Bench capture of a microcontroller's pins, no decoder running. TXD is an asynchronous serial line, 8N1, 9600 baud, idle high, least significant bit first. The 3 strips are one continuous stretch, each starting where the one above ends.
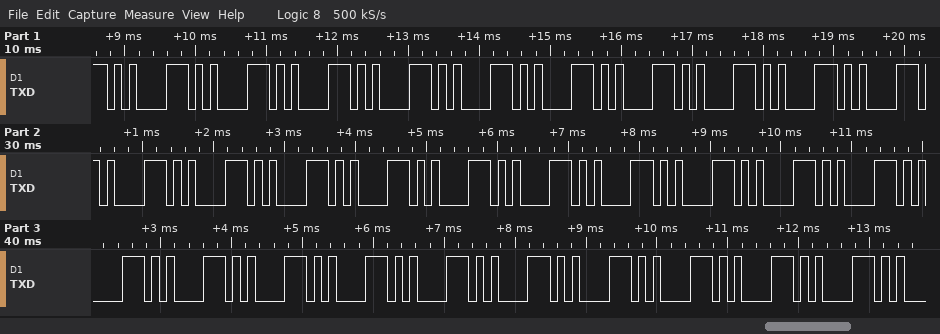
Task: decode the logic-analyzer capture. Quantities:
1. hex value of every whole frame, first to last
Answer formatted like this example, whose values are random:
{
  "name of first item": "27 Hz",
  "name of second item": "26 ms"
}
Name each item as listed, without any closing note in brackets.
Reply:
{
  "hex value of every whole frame, first to last": "85 85 85 85 85 85 85 85 85 85 85 85 85 85 85 85 85 85 85 85 85 85 85 85 85 85 85 85 85 85"
}
